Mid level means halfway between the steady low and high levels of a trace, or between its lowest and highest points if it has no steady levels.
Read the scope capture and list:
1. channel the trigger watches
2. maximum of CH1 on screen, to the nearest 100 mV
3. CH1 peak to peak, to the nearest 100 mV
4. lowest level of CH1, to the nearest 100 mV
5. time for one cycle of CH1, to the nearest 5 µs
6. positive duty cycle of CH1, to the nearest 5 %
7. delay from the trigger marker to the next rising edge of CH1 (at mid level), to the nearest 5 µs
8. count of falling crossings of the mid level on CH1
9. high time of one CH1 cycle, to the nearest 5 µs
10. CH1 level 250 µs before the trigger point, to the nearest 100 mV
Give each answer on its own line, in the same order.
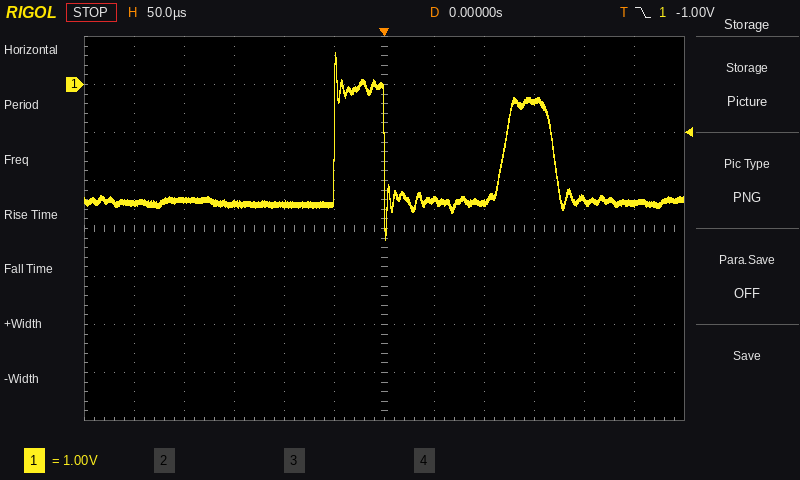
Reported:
CH1
700 mV
3.9 V
-3.2 V
170 µs
30 %
120 µs
2
50 µs
-2.5 V
